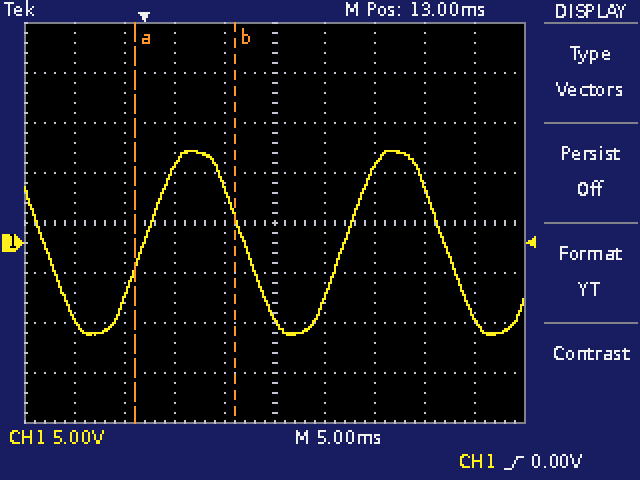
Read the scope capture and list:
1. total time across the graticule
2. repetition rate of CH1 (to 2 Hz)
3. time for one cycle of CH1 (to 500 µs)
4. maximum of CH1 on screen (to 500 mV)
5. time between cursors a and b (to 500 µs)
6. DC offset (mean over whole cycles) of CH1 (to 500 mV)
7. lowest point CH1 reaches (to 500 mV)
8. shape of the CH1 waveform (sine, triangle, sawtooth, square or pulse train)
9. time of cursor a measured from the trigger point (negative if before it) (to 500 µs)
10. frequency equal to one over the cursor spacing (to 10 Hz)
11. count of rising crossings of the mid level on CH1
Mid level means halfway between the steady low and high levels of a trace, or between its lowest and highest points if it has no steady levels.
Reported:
50 ms
50 Hz
20.0 ms
9.0 V
10.0 ms
0.0 V
-9.0 V
sine
-1.0 ms
100 Hz
2
